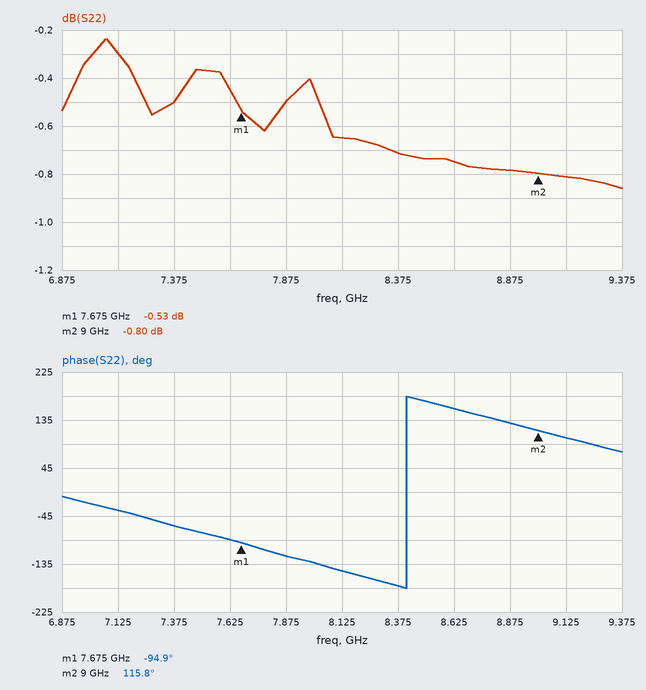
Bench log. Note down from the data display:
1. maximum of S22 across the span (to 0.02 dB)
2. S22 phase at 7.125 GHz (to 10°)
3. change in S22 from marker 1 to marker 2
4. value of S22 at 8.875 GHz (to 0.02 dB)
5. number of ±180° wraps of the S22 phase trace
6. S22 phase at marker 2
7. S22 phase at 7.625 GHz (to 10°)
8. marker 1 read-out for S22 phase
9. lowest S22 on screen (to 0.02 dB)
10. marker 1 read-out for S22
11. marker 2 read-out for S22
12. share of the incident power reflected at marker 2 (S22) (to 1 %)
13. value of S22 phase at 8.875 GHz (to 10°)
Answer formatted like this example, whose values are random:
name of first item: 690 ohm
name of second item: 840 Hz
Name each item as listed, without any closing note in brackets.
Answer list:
maximum of S22 across the span: -0.24 dB
S22 phase at 7.125 GHz: -30°
change in S22 from marker 1 to marker 2: -0.27 dB
value of S22 at 8.875 GHz: -0.78 dB
number of ±180° wraps of the S22 phase trace: 1
S22 phase at marker 2: 115.8°
S22 phase at 7.625 GHz: -90°
marker 1 read-out for S22 phase: -94.9°
lowest S22 on screen: -0.86 dB
marker 1 read-out for S22: -0.53 dB
marker 2 read-out for S22: -0.80 dB
share of the incident power reflected at marker 2 (S22): 83 %
value of S22 phase at 8.875 GHz: 130°
